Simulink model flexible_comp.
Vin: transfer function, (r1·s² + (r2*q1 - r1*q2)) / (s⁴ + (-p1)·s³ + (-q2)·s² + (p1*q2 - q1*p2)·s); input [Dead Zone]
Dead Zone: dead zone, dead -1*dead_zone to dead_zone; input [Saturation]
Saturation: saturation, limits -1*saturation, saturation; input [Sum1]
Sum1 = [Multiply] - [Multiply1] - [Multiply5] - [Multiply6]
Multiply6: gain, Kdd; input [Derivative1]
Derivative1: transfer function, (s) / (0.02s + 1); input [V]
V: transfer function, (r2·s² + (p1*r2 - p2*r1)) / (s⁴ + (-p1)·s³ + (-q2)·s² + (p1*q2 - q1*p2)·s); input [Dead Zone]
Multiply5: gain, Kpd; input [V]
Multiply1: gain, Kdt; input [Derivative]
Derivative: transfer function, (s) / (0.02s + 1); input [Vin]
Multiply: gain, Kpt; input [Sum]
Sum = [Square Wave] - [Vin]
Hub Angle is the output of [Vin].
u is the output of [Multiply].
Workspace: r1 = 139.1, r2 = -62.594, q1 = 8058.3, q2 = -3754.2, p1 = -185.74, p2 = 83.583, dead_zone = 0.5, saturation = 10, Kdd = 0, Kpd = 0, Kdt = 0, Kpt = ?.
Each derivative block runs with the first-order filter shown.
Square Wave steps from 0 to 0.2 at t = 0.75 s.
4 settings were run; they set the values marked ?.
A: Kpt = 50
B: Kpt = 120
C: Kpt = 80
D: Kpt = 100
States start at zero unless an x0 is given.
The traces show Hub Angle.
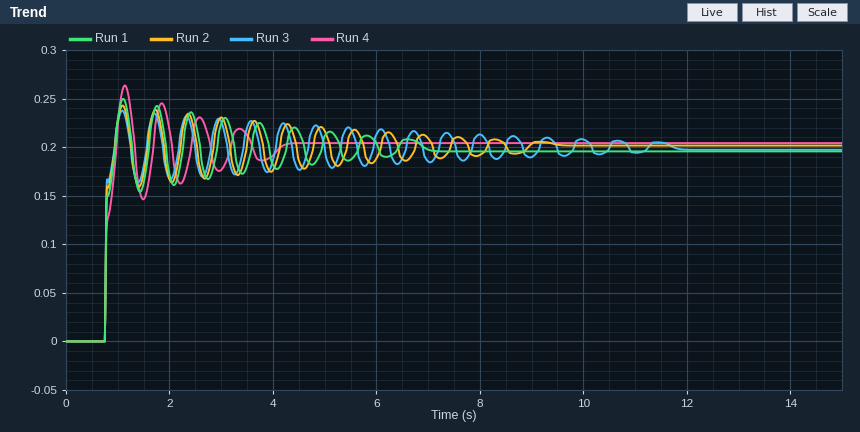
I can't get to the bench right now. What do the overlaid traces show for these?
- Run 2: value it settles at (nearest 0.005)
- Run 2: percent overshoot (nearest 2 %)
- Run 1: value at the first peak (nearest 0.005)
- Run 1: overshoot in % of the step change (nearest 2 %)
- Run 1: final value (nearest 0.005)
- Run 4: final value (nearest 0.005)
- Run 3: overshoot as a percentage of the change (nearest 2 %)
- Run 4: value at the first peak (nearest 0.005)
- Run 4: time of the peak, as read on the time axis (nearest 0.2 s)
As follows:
0.200
20 %
0.250
28 %
0.195
0.205
20 %
0.265
1.2 s
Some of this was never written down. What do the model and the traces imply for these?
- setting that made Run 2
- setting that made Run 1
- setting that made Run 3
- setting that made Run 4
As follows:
D
C
B
A
